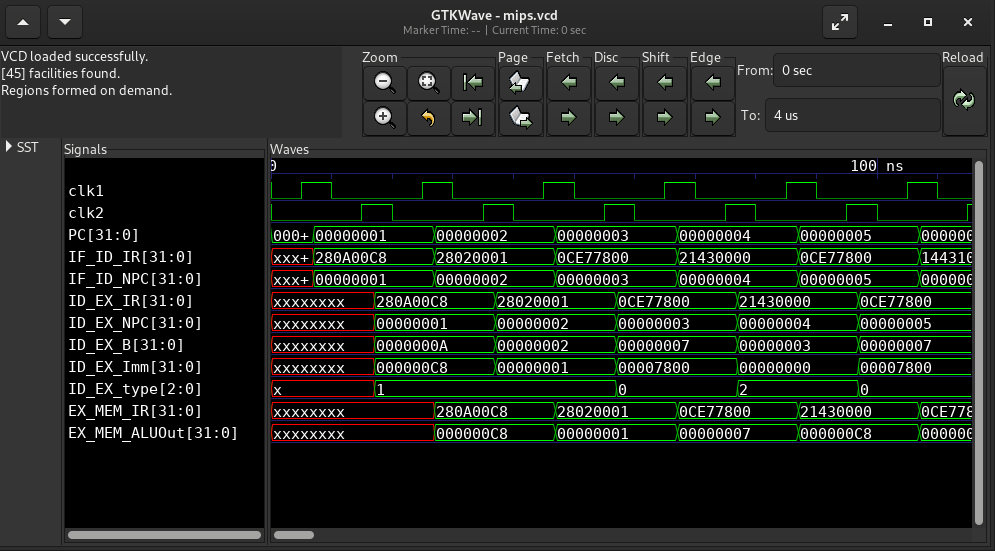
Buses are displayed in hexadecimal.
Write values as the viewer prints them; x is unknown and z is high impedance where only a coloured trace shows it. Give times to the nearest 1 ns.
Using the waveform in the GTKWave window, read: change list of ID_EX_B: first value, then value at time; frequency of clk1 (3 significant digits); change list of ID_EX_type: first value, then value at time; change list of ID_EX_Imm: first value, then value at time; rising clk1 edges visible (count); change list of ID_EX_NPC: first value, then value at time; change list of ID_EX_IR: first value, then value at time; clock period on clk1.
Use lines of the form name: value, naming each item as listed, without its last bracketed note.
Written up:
change list of ID_EX_B: first value, then value at time: xxxxxxxx, 0000000A at 17 ns, 00000002 at 37 ns, 00000007 at 57 ns, 00000003 at 77 ns, 00000007 at 97 ns
frequency of clk1: 50.0 MHz
change list of ID_EX_type: first value, then value at time: x, 1 at 17 ns, 0 at 57 ns, 2 at 77 ns, 0 at 97 ns
change list of ID_EX_Imm: first value, then value at time: xxxxxxxx, 000000C8 at 17 ns, 00000001 at 37 ns, 00007800 at 57 ns, 00000000 at 77 ns, 00007800 at 97 ns
rising clk1 edges visible: 6
change list of ID_EX_NPC: first value, then value at time: xxxxxxxx, 00000001 at 17 ns, 00000002 at 37 ns, 00000003 at 57 ns, 00000004 at 77 ns, 00000005 at 97 ns
change list of ID_EX_IR: first value, then value at time: xxxxxxxx, 280A00C8 at 17 ns, 28020001 at 37 ns, 0CE77800 at 57 ns, 21430000 at 77 ns, 0CE77800 at 97 ns
clock period on clk1: 20 ns
